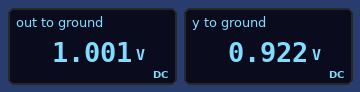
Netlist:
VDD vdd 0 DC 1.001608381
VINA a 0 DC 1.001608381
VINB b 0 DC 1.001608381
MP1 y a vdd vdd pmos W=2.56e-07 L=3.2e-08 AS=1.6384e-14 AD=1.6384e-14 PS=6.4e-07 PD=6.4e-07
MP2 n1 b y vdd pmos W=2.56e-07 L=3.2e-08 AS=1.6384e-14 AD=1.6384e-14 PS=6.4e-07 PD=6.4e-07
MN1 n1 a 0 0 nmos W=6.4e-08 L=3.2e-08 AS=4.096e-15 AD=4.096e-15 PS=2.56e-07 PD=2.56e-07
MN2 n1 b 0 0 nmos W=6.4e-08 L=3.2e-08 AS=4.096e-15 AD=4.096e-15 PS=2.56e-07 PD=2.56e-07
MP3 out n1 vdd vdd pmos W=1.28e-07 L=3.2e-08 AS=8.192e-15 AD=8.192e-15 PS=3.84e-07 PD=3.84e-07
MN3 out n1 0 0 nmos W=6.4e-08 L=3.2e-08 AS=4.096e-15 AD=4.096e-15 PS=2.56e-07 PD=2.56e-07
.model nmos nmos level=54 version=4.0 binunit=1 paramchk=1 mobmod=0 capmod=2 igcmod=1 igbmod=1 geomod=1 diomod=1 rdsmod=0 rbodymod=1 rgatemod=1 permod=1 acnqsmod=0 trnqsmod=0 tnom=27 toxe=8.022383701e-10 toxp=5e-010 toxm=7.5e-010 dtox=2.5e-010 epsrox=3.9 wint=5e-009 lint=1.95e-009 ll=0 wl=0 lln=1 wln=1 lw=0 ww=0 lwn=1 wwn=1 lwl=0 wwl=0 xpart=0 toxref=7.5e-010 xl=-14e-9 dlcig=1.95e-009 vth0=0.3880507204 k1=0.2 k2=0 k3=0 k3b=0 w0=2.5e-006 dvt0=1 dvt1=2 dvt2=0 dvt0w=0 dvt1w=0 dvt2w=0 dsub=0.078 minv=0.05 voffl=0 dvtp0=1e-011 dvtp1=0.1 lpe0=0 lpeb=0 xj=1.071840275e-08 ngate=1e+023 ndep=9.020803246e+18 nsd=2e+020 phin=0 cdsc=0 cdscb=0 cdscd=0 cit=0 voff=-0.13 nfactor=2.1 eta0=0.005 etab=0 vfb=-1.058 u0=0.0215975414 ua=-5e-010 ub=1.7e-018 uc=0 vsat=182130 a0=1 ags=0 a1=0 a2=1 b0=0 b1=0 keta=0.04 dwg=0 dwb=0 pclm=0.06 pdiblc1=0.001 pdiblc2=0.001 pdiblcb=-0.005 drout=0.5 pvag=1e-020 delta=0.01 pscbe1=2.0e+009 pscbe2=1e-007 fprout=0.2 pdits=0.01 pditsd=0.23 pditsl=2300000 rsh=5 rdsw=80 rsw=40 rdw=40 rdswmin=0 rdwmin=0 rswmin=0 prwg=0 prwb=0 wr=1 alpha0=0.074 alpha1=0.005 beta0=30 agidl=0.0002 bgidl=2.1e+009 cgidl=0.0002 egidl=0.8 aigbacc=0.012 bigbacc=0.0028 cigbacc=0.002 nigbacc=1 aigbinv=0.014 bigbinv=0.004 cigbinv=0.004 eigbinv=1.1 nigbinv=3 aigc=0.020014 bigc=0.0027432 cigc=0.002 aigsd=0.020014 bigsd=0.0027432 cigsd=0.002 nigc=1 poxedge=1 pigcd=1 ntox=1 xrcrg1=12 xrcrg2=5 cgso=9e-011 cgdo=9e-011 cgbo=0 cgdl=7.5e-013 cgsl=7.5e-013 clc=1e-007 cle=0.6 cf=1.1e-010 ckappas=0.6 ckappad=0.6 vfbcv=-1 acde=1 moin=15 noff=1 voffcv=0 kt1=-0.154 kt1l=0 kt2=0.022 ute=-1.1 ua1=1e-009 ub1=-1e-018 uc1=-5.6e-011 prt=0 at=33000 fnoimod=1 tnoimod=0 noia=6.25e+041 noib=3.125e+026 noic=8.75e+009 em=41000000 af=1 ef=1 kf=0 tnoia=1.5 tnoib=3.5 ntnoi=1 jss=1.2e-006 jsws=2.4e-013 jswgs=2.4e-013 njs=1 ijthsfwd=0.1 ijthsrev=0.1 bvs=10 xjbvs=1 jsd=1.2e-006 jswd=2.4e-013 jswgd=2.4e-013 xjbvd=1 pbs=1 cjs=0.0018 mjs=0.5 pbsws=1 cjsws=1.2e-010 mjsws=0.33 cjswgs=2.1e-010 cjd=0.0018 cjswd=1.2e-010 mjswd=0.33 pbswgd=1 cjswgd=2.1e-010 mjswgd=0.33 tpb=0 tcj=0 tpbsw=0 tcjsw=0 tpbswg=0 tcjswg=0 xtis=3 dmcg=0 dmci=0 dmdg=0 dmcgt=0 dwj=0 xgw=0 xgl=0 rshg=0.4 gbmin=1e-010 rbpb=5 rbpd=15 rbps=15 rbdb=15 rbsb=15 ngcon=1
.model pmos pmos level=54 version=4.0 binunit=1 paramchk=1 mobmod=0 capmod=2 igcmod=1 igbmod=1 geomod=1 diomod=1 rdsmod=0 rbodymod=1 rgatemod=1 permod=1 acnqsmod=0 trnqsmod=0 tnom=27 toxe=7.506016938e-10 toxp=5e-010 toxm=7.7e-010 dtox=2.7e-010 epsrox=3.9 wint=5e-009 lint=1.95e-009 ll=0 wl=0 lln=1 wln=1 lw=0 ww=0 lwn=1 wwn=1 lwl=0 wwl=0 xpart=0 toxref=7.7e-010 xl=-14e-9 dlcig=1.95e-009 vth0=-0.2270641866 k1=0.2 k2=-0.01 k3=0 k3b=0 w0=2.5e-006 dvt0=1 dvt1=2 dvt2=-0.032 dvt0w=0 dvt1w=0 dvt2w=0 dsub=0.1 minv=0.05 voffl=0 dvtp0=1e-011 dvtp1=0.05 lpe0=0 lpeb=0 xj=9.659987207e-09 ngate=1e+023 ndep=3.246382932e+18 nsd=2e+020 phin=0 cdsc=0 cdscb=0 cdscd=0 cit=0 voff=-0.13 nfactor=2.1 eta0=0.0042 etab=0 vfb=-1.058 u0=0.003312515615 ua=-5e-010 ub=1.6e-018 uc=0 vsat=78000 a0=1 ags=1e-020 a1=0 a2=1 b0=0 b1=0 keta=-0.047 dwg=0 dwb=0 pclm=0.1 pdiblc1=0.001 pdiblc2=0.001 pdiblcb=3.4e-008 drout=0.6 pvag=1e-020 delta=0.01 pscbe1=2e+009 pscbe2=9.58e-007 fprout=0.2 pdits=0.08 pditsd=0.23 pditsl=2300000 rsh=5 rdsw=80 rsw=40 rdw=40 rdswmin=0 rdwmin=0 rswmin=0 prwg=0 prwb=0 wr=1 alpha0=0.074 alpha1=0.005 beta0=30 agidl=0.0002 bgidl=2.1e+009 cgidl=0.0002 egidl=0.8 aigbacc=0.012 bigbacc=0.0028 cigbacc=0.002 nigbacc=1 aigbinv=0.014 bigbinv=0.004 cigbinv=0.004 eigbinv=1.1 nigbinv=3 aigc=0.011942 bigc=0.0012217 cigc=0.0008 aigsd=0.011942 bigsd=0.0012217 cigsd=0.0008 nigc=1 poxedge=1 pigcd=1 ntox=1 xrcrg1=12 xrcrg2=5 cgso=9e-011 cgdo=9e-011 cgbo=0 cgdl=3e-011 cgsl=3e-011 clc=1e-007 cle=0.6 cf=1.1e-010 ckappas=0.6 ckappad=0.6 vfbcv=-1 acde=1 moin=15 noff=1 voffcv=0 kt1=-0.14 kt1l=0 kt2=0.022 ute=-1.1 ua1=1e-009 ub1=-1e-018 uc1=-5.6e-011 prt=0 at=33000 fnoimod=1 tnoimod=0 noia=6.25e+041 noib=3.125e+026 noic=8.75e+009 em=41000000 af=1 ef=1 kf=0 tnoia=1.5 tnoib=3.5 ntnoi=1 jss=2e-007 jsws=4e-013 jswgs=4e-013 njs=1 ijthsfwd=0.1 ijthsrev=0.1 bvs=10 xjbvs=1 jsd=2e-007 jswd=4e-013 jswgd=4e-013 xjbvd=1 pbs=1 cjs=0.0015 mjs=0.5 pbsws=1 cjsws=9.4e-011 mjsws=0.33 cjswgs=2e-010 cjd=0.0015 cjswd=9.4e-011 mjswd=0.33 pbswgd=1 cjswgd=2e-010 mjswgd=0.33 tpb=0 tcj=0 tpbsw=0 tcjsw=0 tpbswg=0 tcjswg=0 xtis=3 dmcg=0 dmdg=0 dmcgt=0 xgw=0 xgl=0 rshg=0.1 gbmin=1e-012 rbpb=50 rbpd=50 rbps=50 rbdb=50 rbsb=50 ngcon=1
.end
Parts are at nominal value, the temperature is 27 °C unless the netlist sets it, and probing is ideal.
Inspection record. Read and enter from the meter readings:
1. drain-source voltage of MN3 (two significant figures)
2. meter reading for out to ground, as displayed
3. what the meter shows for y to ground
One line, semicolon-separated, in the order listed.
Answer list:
1.0 V; 1.001 V; 0.922 V
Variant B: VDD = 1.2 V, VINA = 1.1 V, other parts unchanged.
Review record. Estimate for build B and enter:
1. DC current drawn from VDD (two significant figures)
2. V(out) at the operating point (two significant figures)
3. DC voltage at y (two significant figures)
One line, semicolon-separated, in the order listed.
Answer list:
600 nA; 1.2 V; 1.0 V
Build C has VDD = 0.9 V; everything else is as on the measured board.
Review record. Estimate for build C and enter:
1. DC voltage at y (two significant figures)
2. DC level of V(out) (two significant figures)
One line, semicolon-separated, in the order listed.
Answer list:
850 mV; 900 mV
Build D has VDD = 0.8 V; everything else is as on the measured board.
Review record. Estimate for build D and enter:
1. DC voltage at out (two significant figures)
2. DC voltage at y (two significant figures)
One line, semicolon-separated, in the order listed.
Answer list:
800 mV; 840 mV
